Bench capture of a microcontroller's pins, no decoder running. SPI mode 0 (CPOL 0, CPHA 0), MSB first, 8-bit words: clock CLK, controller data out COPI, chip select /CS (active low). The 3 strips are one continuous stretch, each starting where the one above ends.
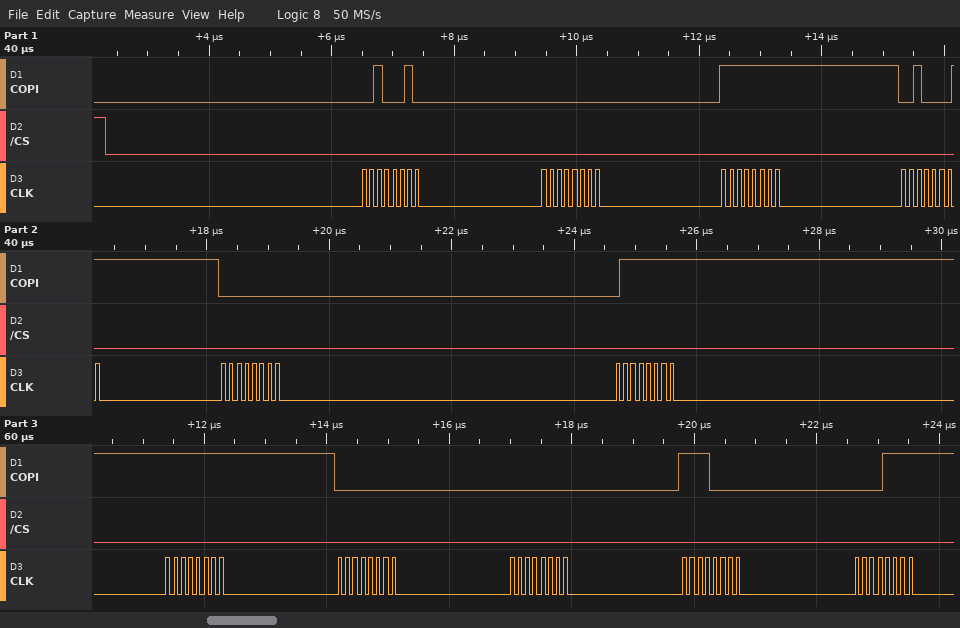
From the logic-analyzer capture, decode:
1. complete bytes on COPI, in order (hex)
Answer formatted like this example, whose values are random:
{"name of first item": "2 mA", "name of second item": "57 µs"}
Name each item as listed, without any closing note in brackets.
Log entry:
{"complete bytes on COPI, in order": "0x22 0x00 0xFF 0x21 0x00 0x7F 0xFF 0x00 0x00 0xF0 0x0F"}
